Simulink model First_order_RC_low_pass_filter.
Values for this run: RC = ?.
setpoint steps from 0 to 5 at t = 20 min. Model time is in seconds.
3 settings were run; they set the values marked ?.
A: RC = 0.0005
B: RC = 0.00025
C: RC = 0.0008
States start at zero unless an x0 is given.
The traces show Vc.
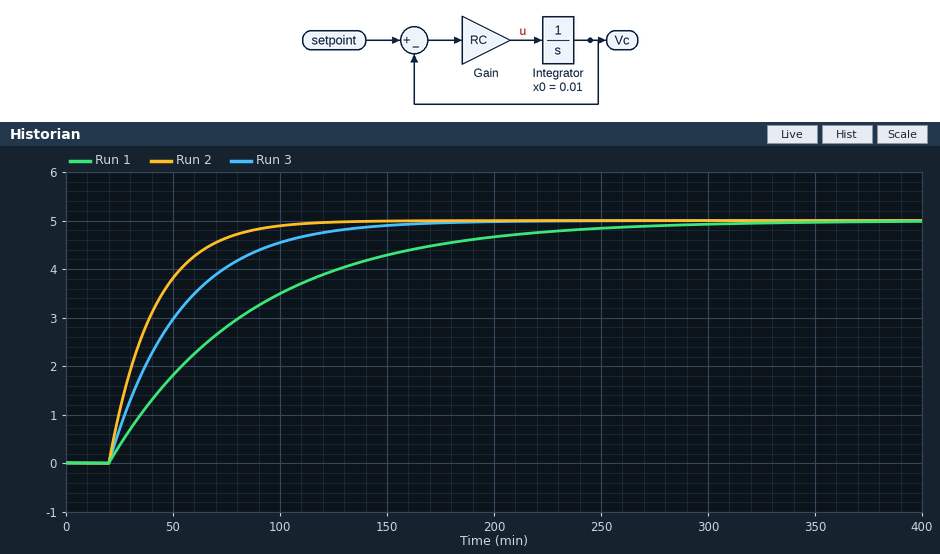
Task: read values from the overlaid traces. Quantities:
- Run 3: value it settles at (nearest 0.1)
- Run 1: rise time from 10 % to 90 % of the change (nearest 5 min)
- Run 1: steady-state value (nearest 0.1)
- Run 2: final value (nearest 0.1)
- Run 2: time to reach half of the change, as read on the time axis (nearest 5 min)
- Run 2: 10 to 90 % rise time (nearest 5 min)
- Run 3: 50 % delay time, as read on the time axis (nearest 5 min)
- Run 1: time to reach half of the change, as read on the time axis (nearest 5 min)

5.0
145 min
5.0
5.0
35 min
45 min
45 min
65 min
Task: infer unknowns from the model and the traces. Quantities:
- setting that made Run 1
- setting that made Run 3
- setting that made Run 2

B
A
C
